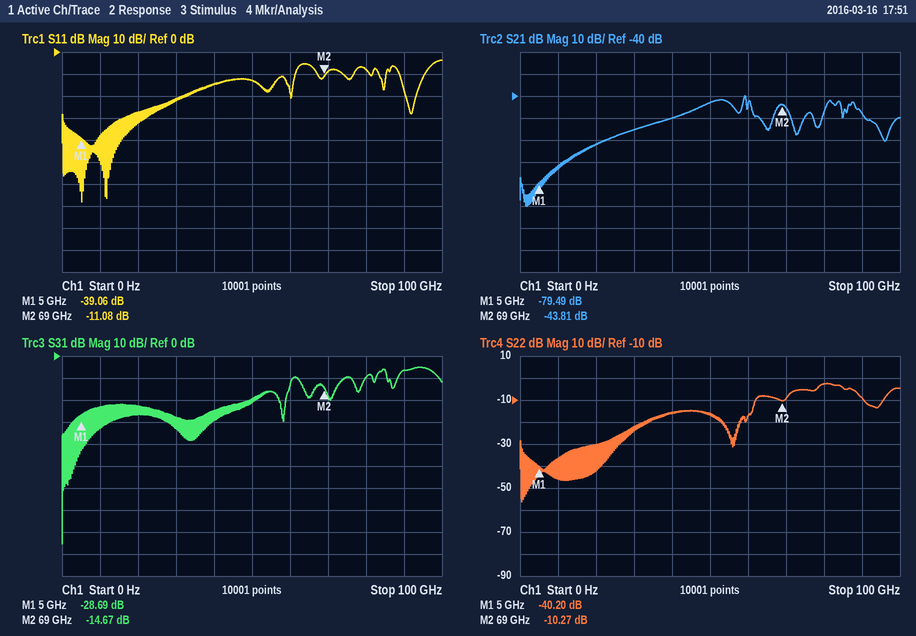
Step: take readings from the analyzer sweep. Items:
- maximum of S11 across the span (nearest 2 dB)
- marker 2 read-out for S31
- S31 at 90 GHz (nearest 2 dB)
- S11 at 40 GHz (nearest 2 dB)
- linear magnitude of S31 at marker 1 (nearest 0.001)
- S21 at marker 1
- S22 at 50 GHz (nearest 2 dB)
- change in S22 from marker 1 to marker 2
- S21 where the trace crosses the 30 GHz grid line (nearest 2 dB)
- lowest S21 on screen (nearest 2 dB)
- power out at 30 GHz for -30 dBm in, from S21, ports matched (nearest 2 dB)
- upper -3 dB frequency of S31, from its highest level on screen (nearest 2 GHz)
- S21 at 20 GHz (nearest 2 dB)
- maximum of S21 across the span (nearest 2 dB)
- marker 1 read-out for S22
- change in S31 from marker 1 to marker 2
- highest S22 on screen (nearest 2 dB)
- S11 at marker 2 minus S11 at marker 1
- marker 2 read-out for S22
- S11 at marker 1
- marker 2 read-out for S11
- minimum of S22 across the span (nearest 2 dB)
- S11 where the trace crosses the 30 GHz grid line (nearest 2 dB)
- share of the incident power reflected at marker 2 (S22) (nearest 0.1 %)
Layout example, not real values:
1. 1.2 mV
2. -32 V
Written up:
1. -4 dB
2. -14.67 dB
3. -6 dB
4. -14 dB
5. 0.037
6. -79.49 dB
7. -16 dB
8. 29.93 dB
9. -56 dB
10. -90 dB
11. -86 dBm
12. 98 GHz
13. -62 dB
14. -40 dB
15. -40.20 dB
16. 14.02 dB
17. -2 dB
18. 27.98 dB
19. -10.27 dB
20. -39.06 dB
21. -11.08 dB
22. -56 dB
23. -22 dB
24. 9.4 %
